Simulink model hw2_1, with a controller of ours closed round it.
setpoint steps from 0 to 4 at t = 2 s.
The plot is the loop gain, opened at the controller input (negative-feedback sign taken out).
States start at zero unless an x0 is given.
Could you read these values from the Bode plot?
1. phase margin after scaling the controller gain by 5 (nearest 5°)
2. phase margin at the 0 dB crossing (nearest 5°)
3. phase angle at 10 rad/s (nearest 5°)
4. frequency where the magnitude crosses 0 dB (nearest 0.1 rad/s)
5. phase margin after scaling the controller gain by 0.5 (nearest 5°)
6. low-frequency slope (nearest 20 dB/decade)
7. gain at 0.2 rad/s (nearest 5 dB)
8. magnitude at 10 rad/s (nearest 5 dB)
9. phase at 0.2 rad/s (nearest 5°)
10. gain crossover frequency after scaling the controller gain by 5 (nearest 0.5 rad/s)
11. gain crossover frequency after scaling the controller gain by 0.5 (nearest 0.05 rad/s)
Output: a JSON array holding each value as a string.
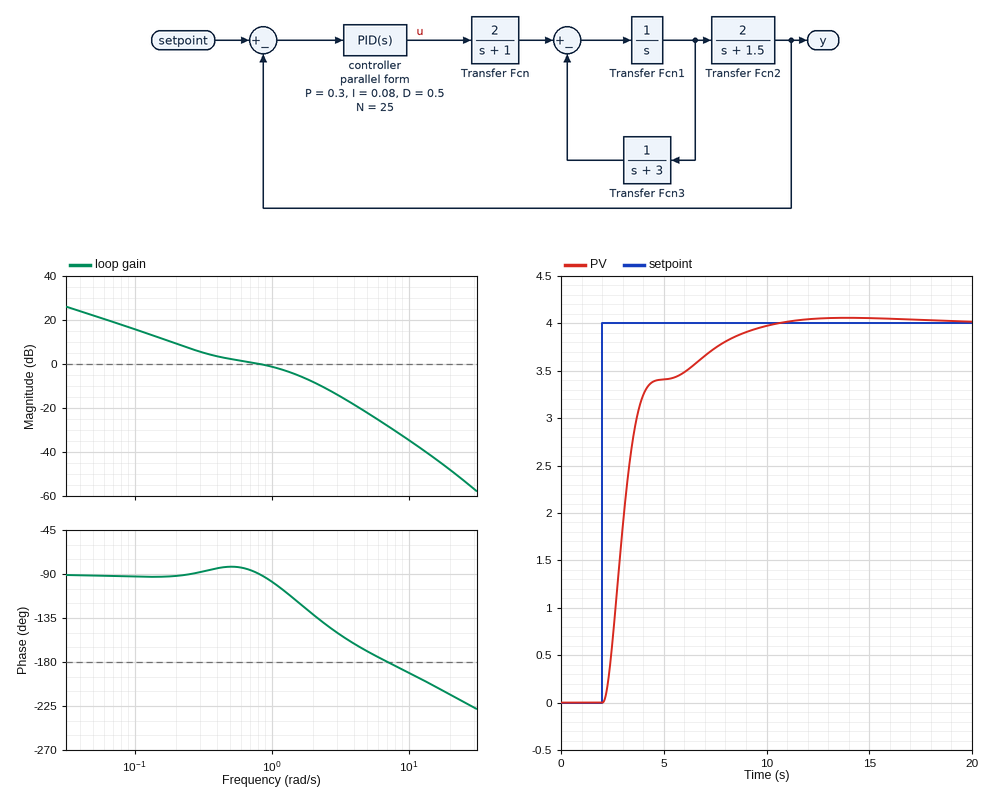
["30°", "90°", "-190°", "0.8 rad/s", "90°", "-20 dB/decade", "10 dB", "-35 dB", "-90°", "3.0 rad/s", "0.30 rad/s"]
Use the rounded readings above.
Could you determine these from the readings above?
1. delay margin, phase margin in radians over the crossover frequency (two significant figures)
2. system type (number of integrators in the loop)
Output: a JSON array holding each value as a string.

["2.0 s", "1"]
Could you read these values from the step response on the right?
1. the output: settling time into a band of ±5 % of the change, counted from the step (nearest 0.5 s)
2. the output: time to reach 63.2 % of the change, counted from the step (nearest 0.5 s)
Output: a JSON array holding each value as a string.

["6.0 s", "1.5 s"]
